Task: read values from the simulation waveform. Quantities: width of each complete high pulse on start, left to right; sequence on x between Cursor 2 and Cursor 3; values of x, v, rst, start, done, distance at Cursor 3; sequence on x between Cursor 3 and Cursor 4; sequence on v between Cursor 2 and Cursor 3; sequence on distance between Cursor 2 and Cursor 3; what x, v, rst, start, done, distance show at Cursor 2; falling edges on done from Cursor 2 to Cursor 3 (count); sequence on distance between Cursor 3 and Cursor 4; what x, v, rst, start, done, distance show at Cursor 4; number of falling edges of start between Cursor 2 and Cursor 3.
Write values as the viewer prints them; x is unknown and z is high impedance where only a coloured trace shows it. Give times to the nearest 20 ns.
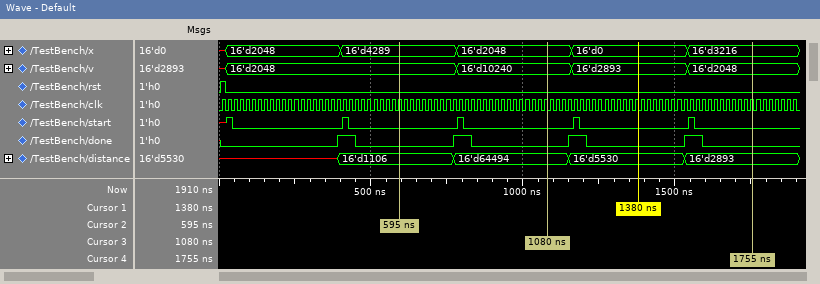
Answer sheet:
20 ns, 20 ns, 20 ns, 20 ns
16'd4289, 16'd2048
x=16'd2048, v=16'd10240, rst=0, start=0, done=0, distance=16'd64494
16'd2048, 16'd0, 16'd3216
16'd2048, 16'd10240
16'd1106, 16'd64494
x=16'd4289, v=16'd2048, rst=0, start=0, done=0, distance=16'd1106
1
16'd64494, 16'd5530, 16'd2893
x=16'd3216, v=16'd2048, rst=0, start=0, done=0, distance=16'd2893
1
